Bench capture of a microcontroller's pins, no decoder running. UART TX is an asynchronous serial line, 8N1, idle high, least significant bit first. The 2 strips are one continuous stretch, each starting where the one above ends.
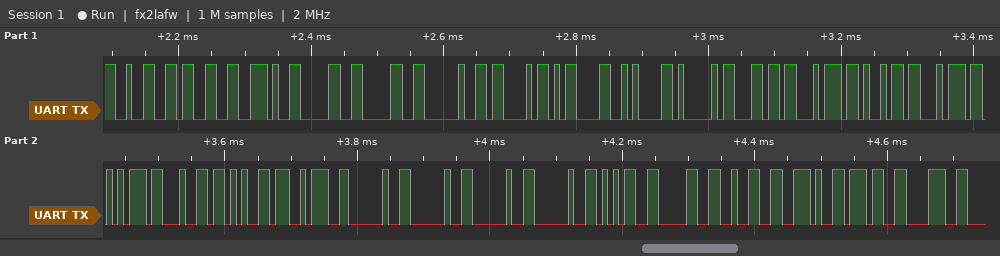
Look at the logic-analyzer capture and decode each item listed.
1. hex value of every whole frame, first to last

32 33 2E 30 30 20 43 0D 0A 41 6C 74 69 74 75 64 65 3A 20 20 20 20 35 30 32 2E 37 38
